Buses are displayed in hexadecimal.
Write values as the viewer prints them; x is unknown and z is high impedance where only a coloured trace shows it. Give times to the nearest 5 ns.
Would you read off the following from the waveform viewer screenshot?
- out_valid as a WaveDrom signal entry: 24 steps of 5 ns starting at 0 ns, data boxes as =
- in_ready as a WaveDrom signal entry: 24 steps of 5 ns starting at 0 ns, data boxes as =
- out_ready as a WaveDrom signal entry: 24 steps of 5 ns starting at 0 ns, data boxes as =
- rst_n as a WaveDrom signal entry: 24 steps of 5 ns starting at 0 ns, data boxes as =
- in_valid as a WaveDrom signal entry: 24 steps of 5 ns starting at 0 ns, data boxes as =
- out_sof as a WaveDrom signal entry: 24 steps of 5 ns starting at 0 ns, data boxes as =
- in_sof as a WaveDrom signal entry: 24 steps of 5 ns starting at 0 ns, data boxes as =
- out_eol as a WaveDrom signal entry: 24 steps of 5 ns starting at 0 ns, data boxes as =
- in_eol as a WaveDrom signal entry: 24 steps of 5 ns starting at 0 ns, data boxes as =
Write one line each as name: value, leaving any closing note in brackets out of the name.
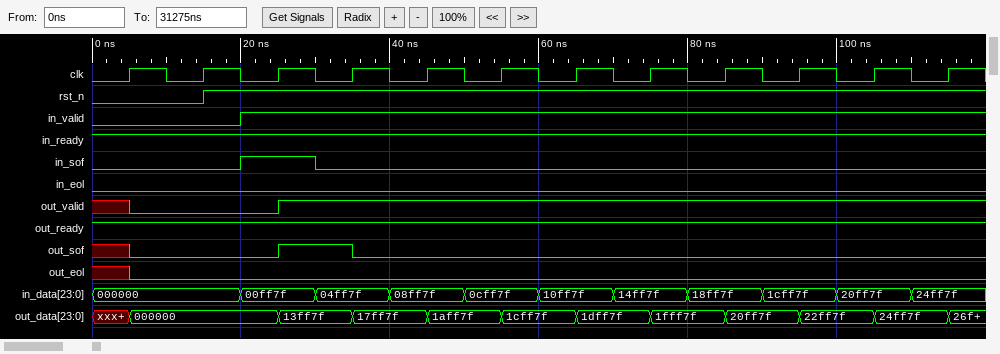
out_valid as a WaveDrom signal entry: 24 steps of 5 ns starting at 0 ns, data boxes as =: {name: 'out_valid', wave: 'x0...1..................'}
in_ready as a WaveDrom signal entry: 24 steps of 5 ns starting at 0 ns, data boxes as =: {name: 'in_ready', wave: '1.......................'}
out_ready as a WaveDrom signal entry: 24 steps of 5 ns starting at 0 ns, data boxes as =: {name: 'out_ready', wave: '1.......................'}
rst_n as a WaveDrom signal entry: 24 steps of 5 ns starting at 0 ns, data boxes as =: {name: 'rst_n', wave: '0..1....................'}
in_valid as a WaveDrom signal entry: 24 steps of 5 ns starting at 0 ns, data boxes as =: {name: 'in_valid', wave: '0...1...................'}
out_sof as a WaveDrom signal entry: 24 steps of 5 ns starting at 0 ns, data boxes as =: {name: 'out_sof', wave: 'x0...1.0................'}
in_sof as a WaveDrom signal entry: 24 steps of 5 ns starting at 0 ns, data boxes as =: {name: 'in_sof', wave: '0...1.0.................'}
out_eol as a WaveDrom signal entry: 24 steps of 5 ns starting at 0 ns, data boxes as =: {name: 'out_eol', wave: 'x0......................'}
in_eol as a WaveDrom signal entry: 24 steps of 5 ns starting at 0 ns, data boxes as =: {name: 'in_eol', wave: '0.......................'}
